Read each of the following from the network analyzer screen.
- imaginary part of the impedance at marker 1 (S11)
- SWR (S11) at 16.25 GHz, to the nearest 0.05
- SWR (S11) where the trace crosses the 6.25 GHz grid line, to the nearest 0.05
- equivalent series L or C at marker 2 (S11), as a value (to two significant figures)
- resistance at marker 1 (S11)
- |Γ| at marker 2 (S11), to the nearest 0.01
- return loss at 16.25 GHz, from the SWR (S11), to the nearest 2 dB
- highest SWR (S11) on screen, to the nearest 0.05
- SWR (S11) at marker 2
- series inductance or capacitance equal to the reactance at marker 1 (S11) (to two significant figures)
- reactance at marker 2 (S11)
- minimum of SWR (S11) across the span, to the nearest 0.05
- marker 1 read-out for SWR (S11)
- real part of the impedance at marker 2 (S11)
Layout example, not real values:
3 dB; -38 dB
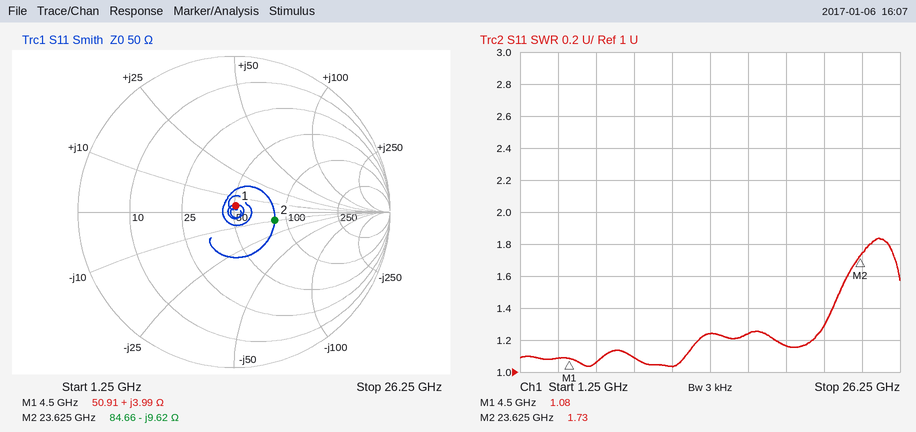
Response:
+3.99 Ω; 1.25; 1.05; 700 fF; 50.91 Ω; 0.27; 20 dB; 1.85; 1.73; 140 pH; -9.62 Ω; 1.05; 1.08; 84.66 Ω
